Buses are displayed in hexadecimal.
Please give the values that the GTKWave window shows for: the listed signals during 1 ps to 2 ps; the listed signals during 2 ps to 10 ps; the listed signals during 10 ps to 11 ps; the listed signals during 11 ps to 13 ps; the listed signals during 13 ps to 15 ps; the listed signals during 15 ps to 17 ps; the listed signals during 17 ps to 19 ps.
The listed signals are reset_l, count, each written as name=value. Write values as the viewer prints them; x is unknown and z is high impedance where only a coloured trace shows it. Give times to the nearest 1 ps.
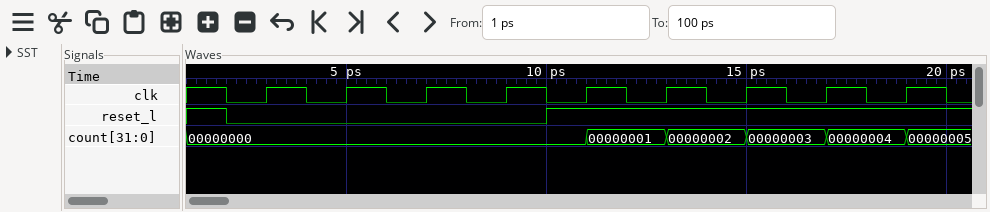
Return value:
reset_l=1, count=00000000
reset_l=0, count=00000000
reset_l=1, count=00000000
reset_l=1, count=00000001
reset_l=1, count=00000002
reset_l=1, count=00000003
reset_l=1, count=00000004
